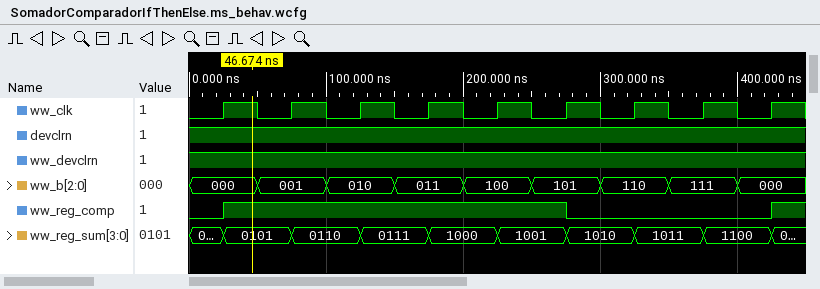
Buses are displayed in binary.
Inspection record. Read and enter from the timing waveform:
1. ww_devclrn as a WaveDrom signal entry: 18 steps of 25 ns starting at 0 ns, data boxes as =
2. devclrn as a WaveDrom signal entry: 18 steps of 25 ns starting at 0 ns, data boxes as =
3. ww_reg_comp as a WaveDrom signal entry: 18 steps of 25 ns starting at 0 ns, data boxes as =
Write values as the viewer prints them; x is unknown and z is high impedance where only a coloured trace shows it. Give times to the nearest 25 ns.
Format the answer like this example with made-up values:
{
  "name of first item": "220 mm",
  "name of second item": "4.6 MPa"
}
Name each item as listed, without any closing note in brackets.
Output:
{
  "ww_devclrn as a WaveDrom signal entry: 18 steps of 25 ns starting at 0 ns, data boxes as =": "{name: 'ww_devclrn', wave: '1.................'}",
  "devclrn as a WaveDrom signal entry: 18 steps of 25 ns starting at 0 ns, data boxes as =": "{name: 'devclrn', wave: '1.................'}",
  "ww_reg_comp as a WaveDrom signal entry: 18 steps of 25 ns starting at 0 ns, data boxes as =": "{name: 'ww_reg_comp', wave: '01.........0.....1'}"
}
